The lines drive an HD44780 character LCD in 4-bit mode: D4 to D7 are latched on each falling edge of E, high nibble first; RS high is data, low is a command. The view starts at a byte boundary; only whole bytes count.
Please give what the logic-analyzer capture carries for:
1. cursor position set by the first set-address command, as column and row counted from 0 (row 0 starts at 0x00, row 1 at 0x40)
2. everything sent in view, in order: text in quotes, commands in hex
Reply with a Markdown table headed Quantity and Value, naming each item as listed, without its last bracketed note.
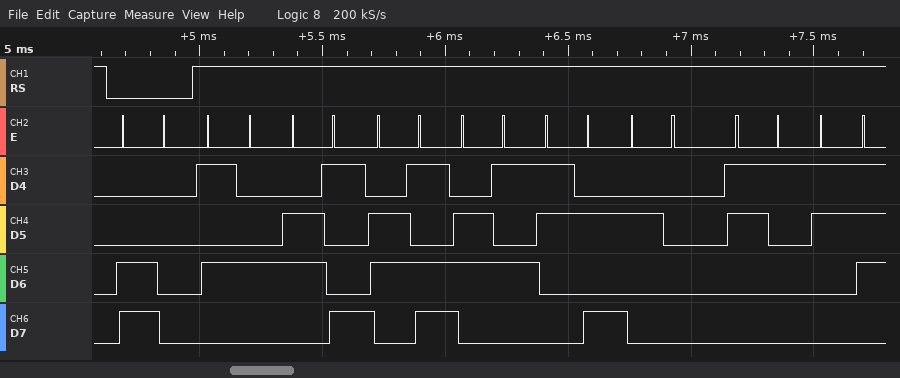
| Quantity | Value |
|---|---|
| cursor position set by the first set-address command, as column and row counted from 0 | column 0, row 1 |
| everything sent in view, in order: text in quotes, commands in hex | 0xC0 "Time: 17" |
